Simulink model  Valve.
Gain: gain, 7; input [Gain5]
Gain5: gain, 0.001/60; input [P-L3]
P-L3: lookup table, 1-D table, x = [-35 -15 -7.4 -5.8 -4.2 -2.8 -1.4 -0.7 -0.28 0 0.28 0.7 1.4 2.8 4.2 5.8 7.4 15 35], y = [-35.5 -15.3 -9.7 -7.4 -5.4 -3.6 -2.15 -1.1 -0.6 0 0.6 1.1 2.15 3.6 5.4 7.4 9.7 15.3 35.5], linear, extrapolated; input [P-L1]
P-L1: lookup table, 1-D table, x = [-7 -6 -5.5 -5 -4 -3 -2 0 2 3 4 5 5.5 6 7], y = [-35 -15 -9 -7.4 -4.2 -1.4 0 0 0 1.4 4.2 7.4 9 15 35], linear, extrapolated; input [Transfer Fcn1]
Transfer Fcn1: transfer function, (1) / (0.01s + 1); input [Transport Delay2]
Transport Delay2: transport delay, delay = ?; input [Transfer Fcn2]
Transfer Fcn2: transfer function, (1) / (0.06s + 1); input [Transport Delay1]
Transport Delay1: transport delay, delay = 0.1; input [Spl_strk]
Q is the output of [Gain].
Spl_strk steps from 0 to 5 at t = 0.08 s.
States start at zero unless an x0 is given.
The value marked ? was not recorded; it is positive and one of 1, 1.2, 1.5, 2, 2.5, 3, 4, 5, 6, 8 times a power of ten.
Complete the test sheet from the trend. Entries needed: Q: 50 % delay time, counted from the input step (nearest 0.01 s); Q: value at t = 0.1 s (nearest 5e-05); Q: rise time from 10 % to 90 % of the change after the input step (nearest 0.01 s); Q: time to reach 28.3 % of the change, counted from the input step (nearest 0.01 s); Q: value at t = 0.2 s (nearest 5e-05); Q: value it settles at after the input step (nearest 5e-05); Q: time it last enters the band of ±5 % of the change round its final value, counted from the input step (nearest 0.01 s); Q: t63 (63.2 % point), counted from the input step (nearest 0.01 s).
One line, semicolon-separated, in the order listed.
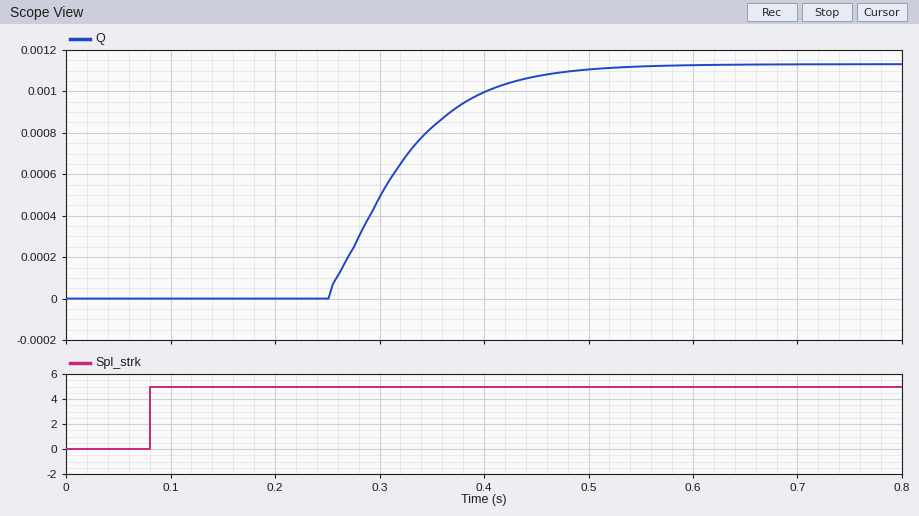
0.23 s; 0.00000; 0.15 s; 0.20 s; 0.00000; 0.00115; 0.37 s; 0.25 s
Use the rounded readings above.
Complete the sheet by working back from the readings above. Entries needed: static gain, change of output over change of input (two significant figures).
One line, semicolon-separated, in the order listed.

0.00023
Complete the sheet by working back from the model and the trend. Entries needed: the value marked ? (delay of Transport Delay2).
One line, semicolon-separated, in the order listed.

0.03
